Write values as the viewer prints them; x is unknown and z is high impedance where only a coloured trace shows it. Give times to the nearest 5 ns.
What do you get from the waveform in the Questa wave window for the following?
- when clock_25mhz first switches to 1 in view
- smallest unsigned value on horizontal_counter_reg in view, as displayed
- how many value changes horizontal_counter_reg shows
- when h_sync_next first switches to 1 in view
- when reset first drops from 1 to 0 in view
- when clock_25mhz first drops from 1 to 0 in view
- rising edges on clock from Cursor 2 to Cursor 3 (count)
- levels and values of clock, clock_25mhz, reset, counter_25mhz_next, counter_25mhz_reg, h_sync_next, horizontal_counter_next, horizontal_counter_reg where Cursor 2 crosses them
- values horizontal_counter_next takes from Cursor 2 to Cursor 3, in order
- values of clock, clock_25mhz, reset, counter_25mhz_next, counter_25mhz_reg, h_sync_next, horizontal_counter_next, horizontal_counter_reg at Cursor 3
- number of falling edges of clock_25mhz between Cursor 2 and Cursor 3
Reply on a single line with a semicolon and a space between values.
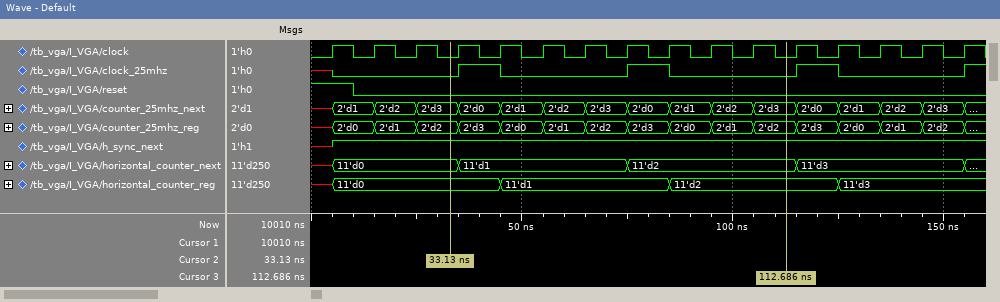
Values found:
35 ns; 11'd0; 4; 5 ns; 10 ns; 45 ns; 8; clock=0, clock_25mhz=0, reset=0, counter_25mhz_next=2'd3, counter_25mhz_reg=2'd2, h_sync_next=1, horizontal_counter_next=11'd0, horizontal_counter_reg=11'd0; 11'd0, 11'd1, 11'd2; clock=0, clock_25mhz=0, reset=0, counter_25mhz_next=2'd3, counter_25mhz_reg=2'd2, h_sync_next=1, horizontal_counter_next=11'd2, horizontal_counter_reg=11'd2; 2
